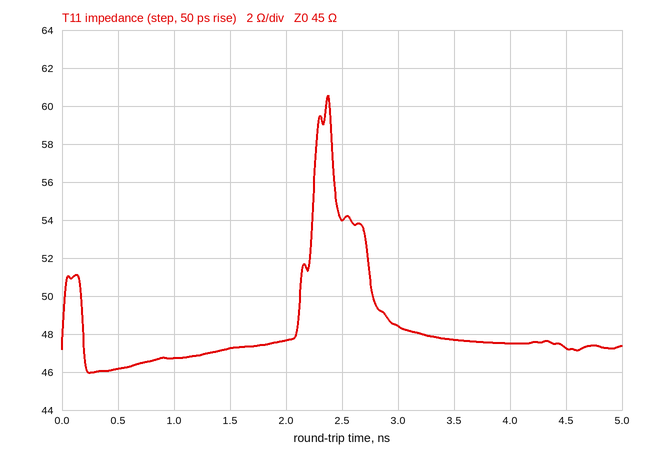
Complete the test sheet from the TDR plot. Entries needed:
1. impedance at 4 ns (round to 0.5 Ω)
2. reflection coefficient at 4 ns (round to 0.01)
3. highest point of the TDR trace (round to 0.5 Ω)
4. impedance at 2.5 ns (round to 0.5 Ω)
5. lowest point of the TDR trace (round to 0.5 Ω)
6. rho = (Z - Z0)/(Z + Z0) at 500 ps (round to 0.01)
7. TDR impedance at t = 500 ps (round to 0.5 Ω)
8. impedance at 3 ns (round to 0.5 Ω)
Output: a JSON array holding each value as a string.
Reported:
["47.5 Ω", "+0.03", "60.5 Ω", "54.0 Ω", "46.0 Ω", "+0.01", "46.0 Ω", "48.5 Ω"]
